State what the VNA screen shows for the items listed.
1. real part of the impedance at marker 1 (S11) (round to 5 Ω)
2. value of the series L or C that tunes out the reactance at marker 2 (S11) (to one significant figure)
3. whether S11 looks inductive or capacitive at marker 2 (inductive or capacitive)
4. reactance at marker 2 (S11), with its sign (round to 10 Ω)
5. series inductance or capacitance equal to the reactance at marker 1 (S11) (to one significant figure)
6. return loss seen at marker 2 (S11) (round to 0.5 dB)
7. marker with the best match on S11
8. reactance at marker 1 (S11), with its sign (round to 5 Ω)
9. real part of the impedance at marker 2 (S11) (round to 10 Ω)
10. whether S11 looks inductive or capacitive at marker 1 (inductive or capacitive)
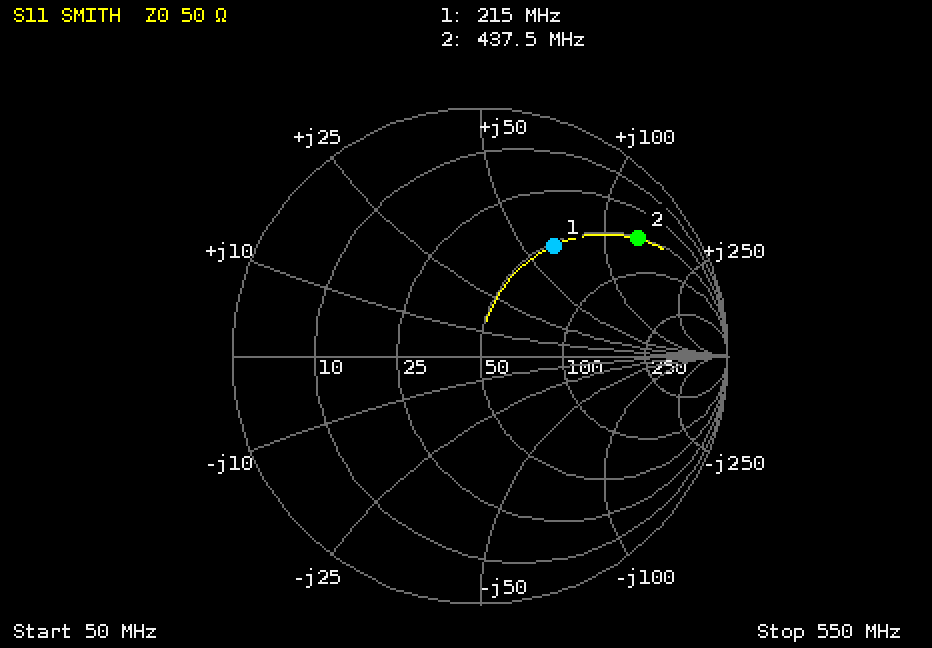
50 Ω
3 pF
inductive
+130 Ω
50 nH
2.0 dB
marker 1
+65 Ω
50 Ω
inductive
